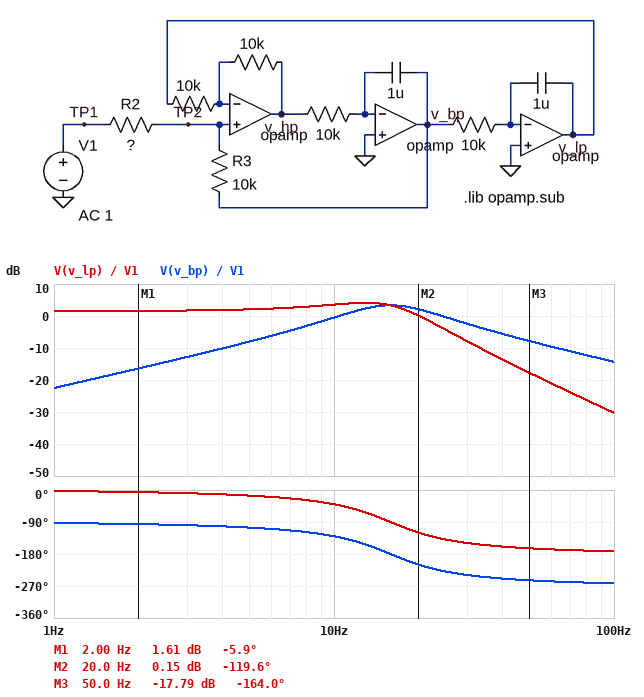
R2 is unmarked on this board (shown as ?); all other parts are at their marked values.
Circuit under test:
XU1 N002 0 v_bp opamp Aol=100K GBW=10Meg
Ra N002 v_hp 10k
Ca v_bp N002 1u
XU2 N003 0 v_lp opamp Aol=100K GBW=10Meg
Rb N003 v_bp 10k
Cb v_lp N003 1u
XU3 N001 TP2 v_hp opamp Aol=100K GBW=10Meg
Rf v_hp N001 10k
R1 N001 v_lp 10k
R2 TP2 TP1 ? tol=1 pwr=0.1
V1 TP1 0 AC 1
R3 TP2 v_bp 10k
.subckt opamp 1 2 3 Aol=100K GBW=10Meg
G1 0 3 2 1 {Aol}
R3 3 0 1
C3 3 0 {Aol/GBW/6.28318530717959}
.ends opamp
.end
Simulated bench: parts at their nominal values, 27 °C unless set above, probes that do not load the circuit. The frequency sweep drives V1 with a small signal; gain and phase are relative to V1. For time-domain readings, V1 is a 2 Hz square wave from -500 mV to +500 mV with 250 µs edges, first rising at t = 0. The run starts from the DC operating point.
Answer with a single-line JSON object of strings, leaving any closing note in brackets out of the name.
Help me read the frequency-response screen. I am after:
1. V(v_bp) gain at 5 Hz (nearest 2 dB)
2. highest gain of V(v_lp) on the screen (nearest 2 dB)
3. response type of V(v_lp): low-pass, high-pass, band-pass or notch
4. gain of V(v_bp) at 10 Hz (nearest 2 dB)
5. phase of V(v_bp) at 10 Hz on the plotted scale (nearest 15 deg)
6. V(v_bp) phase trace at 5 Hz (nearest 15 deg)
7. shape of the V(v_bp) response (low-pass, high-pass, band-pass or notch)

{"V(v_bp) gain at 5 Hz": "-8 dB", "highest gain of V(v_lp) on the screen": "4 dB", "response type of V(v_lp): low-pass, high-pass, band-pass or notch": "low-pass", "gain of V(v_bp) at 10 Hz": "0 dB", "phase of V(v_bp) at 10 Hz on the plotted scale": "-135 deg", "V(v_bp) phase trace at 5 Hz": "-105 deg", "shape of the V(v_bp) response": "band-pass"}
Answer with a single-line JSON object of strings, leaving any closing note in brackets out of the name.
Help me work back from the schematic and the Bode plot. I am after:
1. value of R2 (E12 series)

{"value of R2": "6.8 kΩ"}
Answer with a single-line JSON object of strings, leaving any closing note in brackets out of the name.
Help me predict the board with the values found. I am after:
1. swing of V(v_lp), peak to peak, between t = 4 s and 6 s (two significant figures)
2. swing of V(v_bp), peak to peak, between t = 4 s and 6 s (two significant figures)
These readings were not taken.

{"swing of V(v_lp), peak to peak, between t = 4 s and 6 s": "1.8 V", "swing of V(v_bp), peak to peak, between t = 4 s and 6 s": "1.4 V"}
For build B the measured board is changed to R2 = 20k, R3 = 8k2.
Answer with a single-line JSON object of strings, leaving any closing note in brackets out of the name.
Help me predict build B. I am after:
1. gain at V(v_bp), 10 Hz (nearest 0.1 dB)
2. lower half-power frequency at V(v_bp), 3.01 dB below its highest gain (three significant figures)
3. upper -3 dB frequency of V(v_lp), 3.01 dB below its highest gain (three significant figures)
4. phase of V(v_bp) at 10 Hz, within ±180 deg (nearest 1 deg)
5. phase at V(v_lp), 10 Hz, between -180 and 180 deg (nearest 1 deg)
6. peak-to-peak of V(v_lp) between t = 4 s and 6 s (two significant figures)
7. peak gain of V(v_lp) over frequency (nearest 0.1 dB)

{"gain at V(v_bp), 10 Hz": "-9.4 dB", "lower half-power frequency at V(v_bp), 3.01 dB below its highest gain": "8.22 Hz", "upper -3 dB frequency of V(v_lp), 3.01 dB below its highest gain": "15.9 Hz", "phase of V(v_bp) at 10 Hz, within ±180 deg": "-146 deg", "phase at V(v_lp), 10 Hz, between -180 and 180 deg": "-56 deg", "peak-to-peak of V(v_lp) between t = 4 s and 6 s": "630 mV", "peak gain of V(v_lp) over frequency": "-4.7 dB"}
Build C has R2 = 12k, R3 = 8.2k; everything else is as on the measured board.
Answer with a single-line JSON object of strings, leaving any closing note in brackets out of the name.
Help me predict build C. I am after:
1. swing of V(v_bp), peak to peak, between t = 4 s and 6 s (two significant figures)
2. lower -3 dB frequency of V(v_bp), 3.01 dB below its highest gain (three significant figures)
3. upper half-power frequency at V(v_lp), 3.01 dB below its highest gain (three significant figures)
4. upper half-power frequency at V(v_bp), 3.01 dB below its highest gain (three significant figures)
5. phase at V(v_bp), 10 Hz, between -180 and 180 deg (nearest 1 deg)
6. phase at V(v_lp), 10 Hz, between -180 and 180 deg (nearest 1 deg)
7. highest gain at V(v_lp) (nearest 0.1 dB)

{"swing of V(v_bp), peak to peak, between t = 4 s and 6 s": "820 mV", "lower -3 dB frequency of V(v_bp), 3.01 dB below its highest gain": "9.06 Hz", "upper half-power frequency at V(v_lp), 3.01 dB below its highest gain": "17.8 Hz", "upper half-power frequency at V(v_bp), 3.01 dB below its highest gain": "28.0 Hz", "phase at V(v_bp), 10 Hz, between -180 and 180 deg": "-141 deg", "phase at V(v_lp), 10 Hz, between -180 and 180 deg": "-51 deg", "highest gain at V(v_lp)": "-1.4 dB"}
